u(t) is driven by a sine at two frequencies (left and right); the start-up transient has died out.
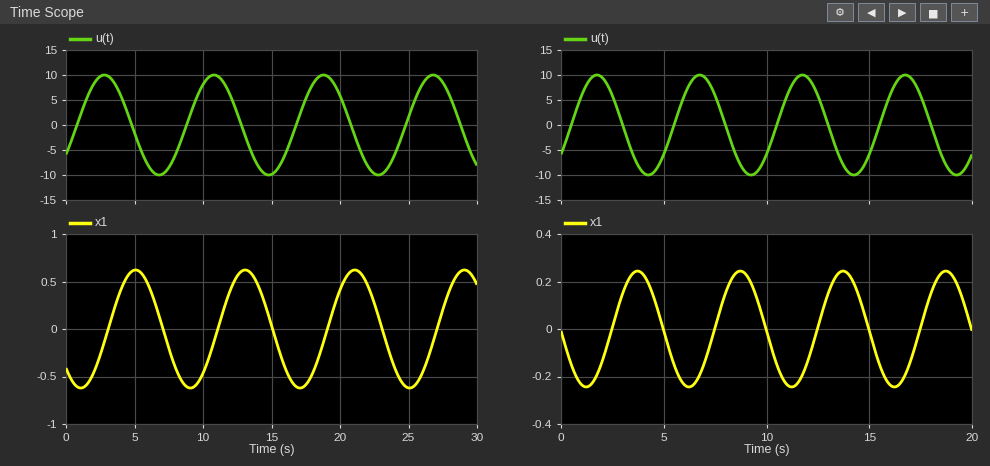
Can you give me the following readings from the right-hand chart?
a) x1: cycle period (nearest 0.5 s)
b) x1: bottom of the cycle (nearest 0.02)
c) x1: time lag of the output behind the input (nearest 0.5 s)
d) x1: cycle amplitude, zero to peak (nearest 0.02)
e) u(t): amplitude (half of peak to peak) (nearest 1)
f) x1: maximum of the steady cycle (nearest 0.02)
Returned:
5.0 s
-0.24
2.0 s
0.24
10
0.24
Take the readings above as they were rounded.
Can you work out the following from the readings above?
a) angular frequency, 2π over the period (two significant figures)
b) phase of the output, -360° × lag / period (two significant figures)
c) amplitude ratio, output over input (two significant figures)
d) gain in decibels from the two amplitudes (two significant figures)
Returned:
1.3 rad/s
-140°
0.024
-32 dB
